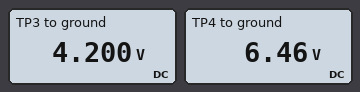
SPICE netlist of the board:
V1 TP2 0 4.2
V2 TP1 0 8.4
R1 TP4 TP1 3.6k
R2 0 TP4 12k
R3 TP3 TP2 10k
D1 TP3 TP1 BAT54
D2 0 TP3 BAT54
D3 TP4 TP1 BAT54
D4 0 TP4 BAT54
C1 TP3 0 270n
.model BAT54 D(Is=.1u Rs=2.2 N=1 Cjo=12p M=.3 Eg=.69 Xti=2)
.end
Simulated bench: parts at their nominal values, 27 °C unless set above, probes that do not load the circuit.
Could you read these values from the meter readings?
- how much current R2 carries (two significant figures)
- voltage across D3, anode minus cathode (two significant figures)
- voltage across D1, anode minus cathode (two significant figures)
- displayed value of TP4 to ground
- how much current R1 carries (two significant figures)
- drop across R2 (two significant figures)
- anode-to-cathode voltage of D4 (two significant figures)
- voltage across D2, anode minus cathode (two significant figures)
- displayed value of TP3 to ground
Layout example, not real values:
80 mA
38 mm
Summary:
540 µA
-1.9 V
-4.2 V
6.46 V
540 µA
6.5 V
-6.5 V
-4.2 V
4.200 V
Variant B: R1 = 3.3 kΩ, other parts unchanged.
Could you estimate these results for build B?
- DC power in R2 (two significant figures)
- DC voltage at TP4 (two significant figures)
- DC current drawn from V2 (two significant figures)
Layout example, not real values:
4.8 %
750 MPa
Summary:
3.6 mW
6.6 V
550 µA
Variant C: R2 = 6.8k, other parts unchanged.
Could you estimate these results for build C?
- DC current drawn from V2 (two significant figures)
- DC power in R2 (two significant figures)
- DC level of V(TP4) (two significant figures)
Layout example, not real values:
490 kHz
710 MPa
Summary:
810 µA
4.4 mW
5.5 V
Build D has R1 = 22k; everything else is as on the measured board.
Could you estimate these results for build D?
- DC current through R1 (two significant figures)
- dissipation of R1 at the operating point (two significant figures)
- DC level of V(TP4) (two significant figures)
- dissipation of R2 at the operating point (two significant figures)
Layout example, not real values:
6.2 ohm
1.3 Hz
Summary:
250 µA
1.3 mW
3.0 V
730 µW
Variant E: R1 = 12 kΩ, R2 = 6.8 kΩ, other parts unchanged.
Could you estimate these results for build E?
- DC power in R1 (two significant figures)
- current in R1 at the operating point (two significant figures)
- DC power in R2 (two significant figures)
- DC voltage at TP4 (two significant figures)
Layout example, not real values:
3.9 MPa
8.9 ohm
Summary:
2.4 mW
450 µA
1.4 mW
3.0 V
